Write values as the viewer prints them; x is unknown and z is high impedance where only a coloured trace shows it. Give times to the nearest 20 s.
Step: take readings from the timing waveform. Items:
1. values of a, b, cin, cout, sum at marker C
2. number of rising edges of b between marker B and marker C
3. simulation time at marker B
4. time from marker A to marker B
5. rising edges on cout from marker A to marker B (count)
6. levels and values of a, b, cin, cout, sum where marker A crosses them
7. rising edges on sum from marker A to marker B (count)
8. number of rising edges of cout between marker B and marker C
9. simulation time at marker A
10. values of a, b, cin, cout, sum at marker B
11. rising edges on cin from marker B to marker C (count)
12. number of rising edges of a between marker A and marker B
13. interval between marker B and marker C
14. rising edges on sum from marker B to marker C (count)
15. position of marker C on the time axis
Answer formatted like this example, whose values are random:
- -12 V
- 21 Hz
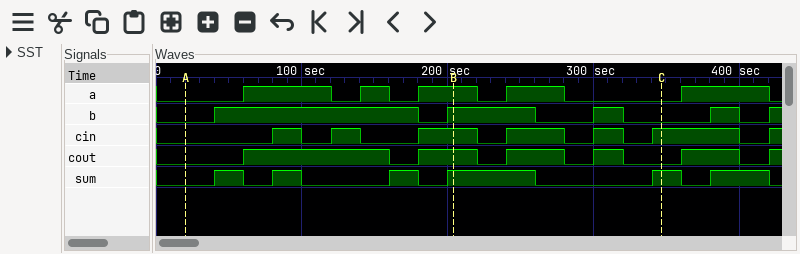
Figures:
- a=0, b=0, cin=1, cout=0, sum=1
- 1
- 200 s
- 180 s
- 2
- a=0, b=0, cin=0, cout=0, sum=0
- 4
- 2
- 20 s
- a=1, b=1, cin=1, cout=1, sum=1
- 3
- 3
- 140 s
- 1
- 340 s
